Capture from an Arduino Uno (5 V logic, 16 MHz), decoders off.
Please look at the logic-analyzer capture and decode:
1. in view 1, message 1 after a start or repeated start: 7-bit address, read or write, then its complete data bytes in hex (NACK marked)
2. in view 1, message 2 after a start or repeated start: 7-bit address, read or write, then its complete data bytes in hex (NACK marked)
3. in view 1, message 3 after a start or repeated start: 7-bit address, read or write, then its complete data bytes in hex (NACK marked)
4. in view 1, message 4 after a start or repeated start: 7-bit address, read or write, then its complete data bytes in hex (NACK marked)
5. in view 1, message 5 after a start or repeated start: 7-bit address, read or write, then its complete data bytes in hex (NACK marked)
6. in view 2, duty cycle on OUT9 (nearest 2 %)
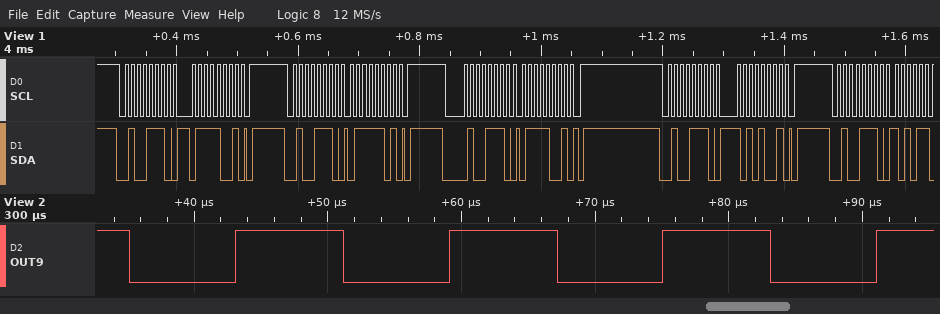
0x27 write: 79
0x27 write: 7D
0x27 write: 79
0x27 write: A9
0x27 write
50 %
